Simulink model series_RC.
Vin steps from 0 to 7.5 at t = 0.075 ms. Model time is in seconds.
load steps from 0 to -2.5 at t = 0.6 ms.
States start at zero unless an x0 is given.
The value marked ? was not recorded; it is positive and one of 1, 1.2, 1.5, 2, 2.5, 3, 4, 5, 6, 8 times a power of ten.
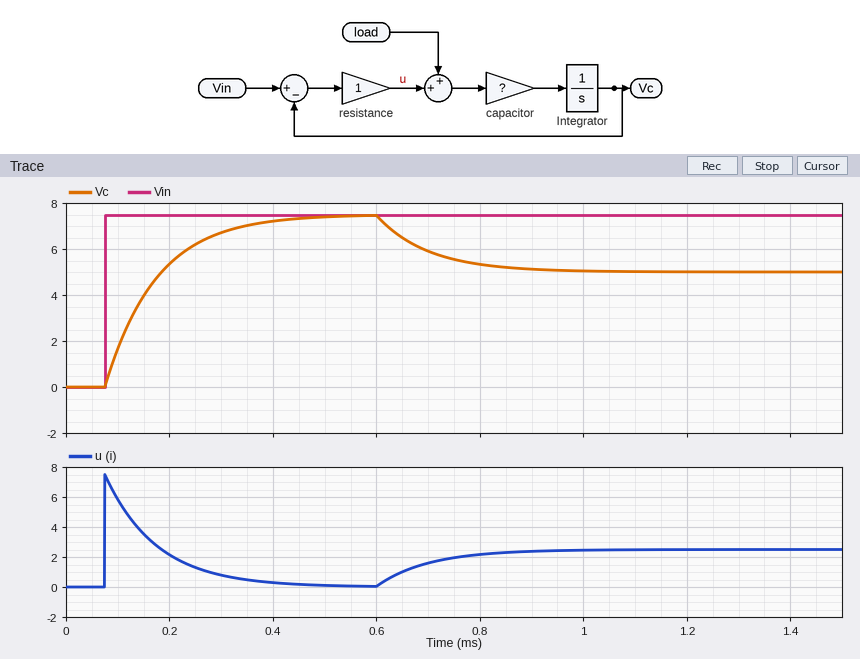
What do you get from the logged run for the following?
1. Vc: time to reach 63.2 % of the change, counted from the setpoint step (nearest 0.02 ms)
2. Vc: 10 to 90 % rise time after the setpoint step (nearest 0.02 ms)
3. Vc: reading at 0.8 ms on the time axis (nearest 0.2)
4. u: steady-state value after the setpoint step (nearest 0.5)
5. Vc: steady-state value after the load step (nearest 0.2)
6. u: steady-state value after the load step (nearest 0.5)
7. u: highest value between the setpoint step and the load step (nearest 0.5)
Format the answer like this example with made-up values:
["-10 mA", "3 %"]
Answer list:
["0.10 ms", "0.22 ms", "5.4", "0.0", "5.0", "2.5", "7.5"]
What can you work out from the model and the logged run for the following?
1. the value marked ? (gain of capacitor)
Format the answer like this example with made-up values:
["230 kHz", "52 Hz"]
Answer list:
["10000"]
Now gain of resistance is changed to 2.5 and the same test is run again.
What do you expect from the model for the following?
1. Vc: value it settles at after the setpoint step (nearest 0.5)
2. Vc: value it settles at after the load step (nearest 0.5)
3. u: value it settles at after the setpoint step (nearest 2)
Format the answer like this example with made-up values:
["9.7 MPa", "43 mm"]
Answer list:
["7.5", "6.5", "0"]
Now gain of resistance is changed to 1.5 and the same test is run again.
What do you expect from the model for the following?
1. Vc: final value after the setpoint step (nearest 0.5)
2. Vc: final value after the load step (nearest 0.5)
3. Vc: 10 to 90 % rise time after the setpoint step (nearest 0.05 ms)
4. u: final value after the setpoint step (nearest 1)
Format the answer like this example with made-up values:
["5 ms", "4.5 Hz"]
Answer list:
["7.5", "6.0", "0.15 ms", "0"]
